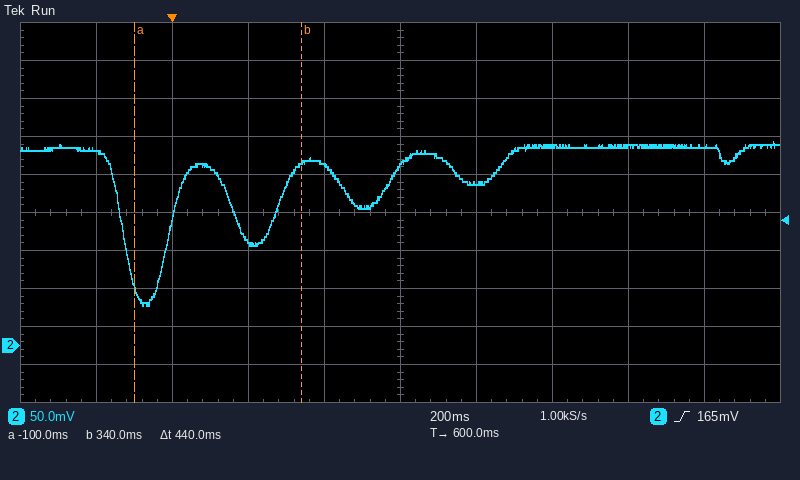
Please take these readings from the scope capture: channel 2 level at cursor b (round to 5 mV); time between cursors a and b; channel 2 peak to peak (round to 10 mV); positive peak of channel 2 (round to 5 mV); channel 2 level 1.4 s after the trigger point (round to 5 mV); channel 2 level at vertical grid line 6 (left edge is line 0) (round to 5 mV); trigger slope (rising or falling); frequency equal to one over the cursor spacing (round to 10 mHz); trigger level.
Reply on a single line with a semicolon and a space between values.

240 mV; 440 ms; 220 mV; 270 mV; 260 mV; 215 mV; rising; 2.27 Hz; 165 mV
